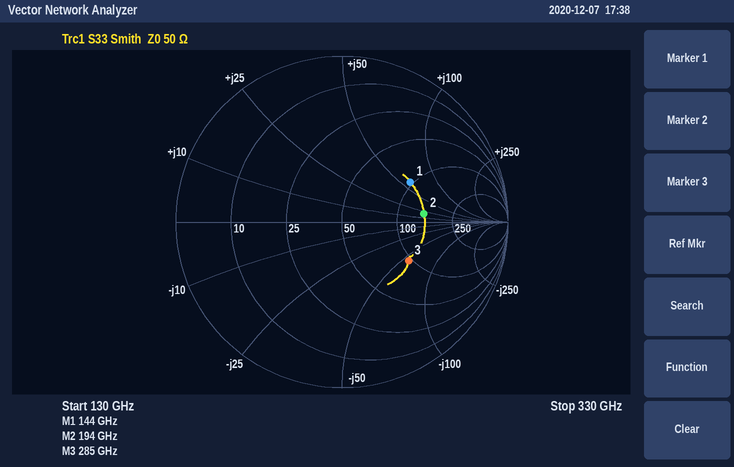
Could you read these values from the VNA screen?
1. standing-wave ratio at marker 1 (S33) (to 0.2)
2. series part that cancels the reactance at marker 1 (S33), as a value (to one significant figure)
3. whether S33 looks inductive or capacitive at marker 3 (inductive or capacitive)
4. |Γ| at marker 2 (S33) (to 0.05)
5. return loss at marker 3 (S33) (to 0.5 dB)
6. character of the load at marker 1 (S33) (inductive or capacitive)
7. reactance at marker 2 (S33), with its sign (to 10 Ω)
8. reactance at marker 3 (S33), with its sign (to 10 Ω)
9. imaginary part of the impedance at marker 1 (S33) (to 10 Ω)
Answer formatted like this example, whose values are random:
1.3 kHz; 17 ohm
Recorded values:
2.8; 20 fF; capacitive; 0.50; 6.5 dB; inductive; +20 Ω; -60 Ω; +60 Ω
